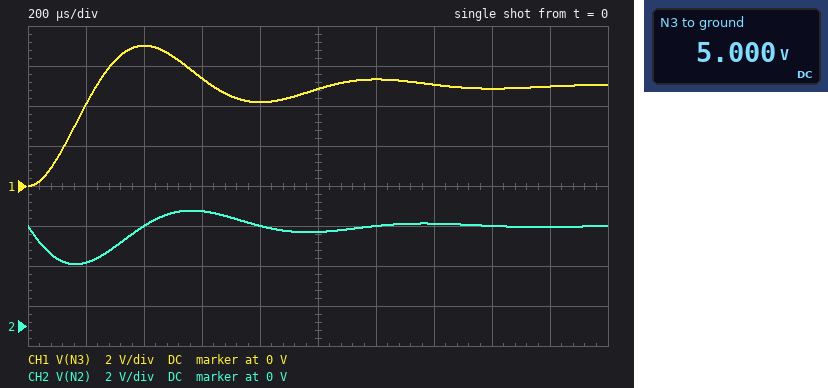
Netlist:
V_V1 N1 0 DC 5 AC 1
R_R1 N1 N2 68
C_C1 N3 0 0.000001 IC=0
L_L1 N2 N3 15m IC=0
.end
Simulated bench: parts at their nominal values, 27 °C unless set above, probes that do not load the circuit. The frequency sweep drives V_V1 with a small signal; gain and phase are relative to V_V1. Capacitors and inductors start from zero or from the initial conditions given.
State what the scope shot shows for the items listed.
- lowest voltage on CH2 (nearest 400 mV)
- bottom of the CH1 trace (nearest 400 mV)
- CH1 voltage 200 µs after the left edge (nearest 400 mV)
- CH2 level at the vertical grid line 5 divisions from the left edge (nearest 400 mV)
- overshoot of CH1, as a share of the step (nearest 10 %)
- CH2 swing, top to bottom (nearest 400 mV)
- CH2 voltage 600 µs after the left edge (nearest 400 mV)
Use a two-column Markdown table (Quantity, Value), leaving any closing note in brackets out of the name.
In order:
| Quantity | Value |
|---|---|
| lowest voltage on CH2 | 3.2 V |
| bottom of the CH1 trace | 0 V |
| CH1 voltage 200 µs after the left edge | 4.0 V |
| CH2 level at the vertical grid line 5 divisions from the left edge | 4.8 V |
| overshoot of CH1, as a share of the step | 40 % |
| CH2 swing, top to bottom | 2.8 V |
| CH2 voltage 600 µs after the left edge | 5.6 V |
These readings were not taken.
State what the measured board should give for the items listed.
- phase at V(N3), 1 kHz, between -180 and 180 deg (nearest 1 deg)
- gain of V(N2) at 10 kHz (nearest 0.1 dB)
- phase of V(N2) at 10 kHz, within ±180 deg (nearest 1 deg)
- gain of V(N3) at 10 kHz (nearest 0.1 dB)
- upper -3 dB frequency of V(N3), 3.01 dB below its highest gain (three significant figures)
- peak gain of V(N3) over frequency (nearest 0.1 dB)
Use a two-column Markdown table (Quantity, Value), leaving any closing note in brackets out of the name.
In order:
| Quantity | Value |
|---|---|
| phase at V(N3), 1 kHz, between -180 and 180 deg | -46 deg |
| gain of V(N2) at 10 kHz | 0 dB |
| phase of V(N2) at 10 kHz, within ±180 deg | 4 deg |
| gain of V(N3) at 10 kHz | -35.3 dB |
| upper -3 dB frequency of V(N3), 3.01 dB below its highest gain | 1.53 kHz |
| peak gain of V(N3) over frequency | 5.5 dB |
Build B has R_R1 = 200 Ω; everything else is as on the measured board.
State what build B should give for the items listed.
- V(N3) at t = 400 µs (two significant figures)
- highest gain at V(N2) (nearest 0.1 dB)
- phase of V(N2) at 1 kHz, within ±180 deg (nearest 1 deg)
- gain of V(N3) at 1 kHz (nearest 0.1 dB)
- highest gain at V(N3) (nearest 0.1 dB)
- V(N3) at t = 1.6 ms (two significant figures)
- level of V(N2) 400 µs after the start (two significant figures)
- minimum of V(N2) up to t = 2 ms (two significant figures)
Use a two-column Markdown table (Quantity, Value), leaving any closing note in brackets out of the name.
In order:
| Quantity | Value |
|---|---|
| V(N3) at t = 400 µs | 4.6 V |
| highest gain at V(N2) | 0 dB |
| phase of V(N2) at 1 kHz, within ±180 deg | -72 deg |
| gain of V(N3) at 1 kHz | -2.4 dB |
| highest gain at V(N3) | 0 dB |
| V(N3) at t = 1.6 ms | 5.0 V |
| level of V(N2) 400 µs after the start | 4.1 V |
| minimum of V(N2) up to t = 2 ms | 1.6 V |
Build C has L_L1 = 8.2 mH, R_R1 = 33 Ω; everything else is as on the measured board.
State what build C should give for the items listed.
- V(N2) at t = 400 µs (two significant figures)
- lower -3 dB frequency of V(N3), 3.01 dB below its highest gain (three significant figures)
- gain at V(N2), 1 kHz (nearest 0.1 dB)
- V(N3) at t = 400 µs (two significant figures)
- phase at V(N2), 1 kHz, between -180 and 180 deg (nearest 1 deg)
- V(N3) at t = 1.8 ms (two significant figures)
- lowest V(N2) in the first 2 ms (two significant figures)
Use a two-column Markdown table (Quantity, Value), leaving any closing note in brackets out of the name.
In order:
| Quantity | Value |
|---|---|
| V(N2) at t = 400 µs | 5.8 V |
| lower -3 dB frequency of V(N3), 3.01 dB below its highest gain | 1.33 kHz |
| gain at V(N2), 1 kHz | -0.4 dB |
| V(N3) at t = 400 µs | 6.2 V |
| phase at V(N2), 1 kHz, between -180 and 180 deg | -17 deg |
| V(N3) at t = 1.8 ms | 4.9 V |
| lowest V(N2) in the first 2 ms | 3.6 V |
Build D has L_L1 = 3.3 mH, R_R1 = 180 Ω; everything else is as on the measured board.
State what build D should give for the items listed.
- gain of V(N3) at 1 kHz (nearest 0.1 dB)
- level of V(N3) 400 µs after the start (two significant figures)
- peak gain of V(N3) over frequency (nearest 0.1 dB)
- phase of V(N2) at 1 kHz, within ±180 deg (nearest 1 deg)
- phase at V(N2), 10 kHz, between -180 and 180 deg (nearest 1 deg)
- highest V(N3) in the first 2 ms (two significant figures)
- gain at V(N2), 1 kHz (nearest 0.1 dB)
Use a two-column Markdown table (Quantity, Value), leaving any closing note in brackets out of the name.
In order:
| Quantity | Value |
|---|---|
| gain of V(N3) at 1 kHz | -3.1 dB |
| level of V(N3) 400 µs after the start | 4.5 V |
| peak gain of V(N3) over frequency | 0 dB |
| phase of V(N2) at 1 kHz, within ±180 deg | -52 deg |
| phase at V(N2), 10 kHz, between -180 and 180 deg | 43 deg |
| highest V(N3) in the first 2 ms | 5.0 V |
| gain at V(N2), 1 kHz | -4.3 dB |
